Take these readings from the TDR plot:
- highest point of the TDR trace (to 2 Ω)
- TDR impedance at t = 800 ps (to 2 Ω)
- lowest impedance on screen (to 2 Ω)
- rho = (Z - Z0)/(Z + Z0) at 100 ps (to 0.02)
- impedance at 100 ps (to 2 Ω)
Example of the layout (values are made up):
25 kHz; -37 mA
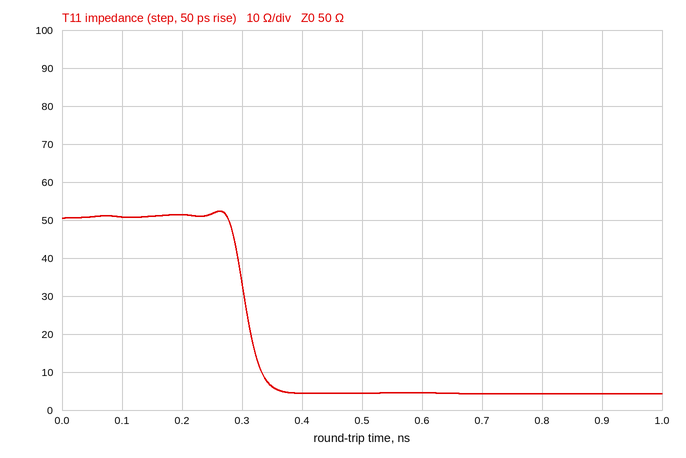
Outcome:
52 Ω; 4 Ω; 4 Ω; 0.00; 50 Ω
